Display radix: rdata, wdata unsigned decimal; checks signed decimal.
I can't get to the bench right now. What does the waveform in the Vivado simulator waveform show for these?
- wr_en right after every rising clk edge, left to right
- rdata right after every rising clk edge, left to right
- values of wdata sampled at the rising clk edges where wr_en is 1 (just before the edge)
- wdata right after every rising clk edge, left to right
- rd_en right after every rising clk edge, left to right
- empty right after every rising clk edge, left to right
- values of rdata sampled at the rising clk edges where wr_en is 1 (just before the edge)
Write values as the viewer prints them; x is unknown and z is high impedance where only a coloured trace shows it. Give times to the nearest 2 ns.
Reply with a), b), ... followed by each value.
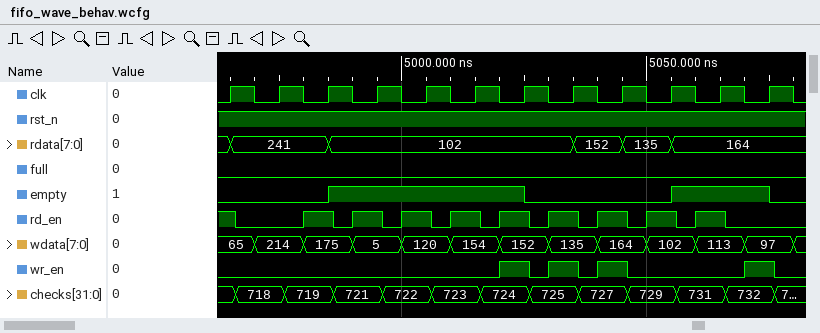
a) 0 0 0 0 0 0 1 1 1 0 0 1
b) 241, 241, 102, 102, 102, 102, 102, 152, 135, 164, 164, 164
c) 152, 135, 164, 97
d) 65, 214, 175, 5, 120, 154, 152, 135, 164, 102, 113, 97
e) 1 0 1 1 1 1 1 1 1 1 1 0
f) 0 0 1 1 1 1 0 0 0 1 1 0
g) 102, 102, 152, 164
